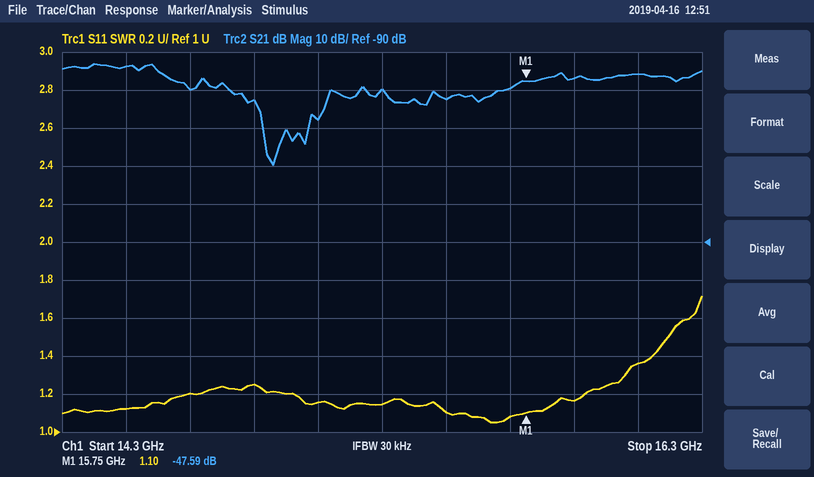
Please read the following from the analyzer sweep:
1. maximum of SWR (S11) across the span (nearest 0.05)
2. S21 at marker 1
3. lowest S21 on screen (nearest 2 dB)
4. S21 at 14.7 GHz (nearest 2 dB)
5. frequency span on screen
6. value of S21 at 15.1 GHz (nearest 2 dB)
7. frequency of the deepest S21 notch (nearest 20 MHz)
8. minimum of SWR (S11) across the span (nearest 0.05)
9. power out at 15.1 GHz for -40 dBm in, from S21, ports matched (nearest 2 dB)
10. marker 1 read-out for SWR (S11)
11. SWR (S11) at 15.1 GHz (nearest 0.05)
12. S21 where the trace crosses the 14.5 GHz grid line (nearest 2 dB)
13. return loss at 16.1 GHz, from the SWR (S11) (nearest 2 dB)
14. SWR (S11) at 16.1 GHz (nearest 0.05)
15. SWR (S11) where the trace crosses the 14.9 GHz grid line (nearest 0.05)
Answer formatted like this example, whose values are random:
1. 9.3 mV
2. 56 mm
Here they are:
1. 1.70
2. -47.59 dB
3. -70 dB
4. -50 dB
5. 2 GHz
6. -58 dB
7. 14.96 GHz
8. 1.05
9. -98 dBm
10. 1.10
11. 1.15
12. -44 dB
13. 16 dB
14. 1.35
15. 1.25
